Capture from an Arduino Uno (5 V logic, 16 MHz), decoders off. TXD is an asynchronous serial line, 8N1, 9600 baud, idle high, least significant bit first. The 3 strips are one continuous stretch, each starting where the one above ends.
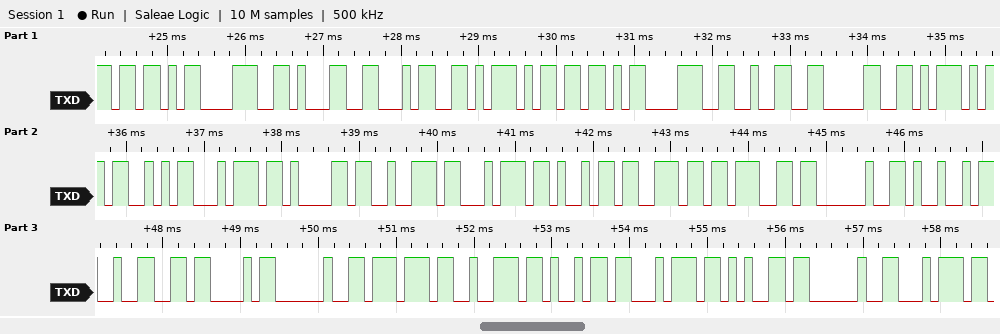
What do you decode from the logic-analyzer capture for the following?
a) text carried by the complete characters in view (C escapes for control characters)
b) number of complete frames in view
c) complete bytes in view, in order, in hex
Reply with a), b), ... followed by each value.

a) "[814][820]Starting I2C write t"
b) 30
c) 5B 38 31 34 5D 5B 38 32 30 5D 53 74 61 72 74 69 6E 67 20 49 32 43 20 77 72 69 74 65 20 74
